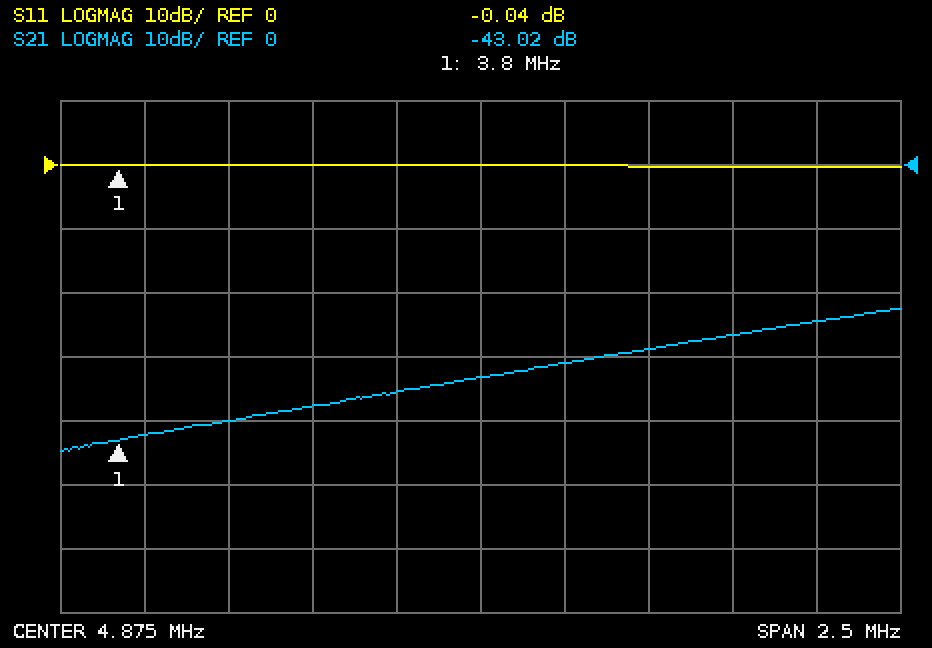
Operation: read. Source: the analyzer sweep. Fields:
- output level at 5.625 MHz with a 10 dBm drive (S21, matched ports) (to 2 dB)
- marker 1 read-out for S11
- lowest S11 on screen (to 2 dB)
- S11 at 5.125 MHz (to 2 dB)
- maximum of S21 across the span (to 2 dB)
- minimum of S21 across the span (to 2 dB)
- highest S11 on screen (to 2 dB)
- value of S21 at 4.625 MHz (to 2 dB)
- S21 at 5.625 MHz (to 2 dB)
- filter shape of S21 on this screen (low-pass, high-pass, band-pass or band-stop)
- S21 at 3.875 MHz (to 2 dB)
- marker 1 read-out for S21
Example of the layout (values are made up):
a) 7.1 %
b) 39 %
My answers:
a) -16 dBm
b) -0.04 dB
c) 0 dB
d) 0 dB
e) -22 dB
f) -44 dB
g) 0 dB
h) -36 dB
i) -26 dB
j) high-pass
k) -42 dB
l) -43.02 dB
